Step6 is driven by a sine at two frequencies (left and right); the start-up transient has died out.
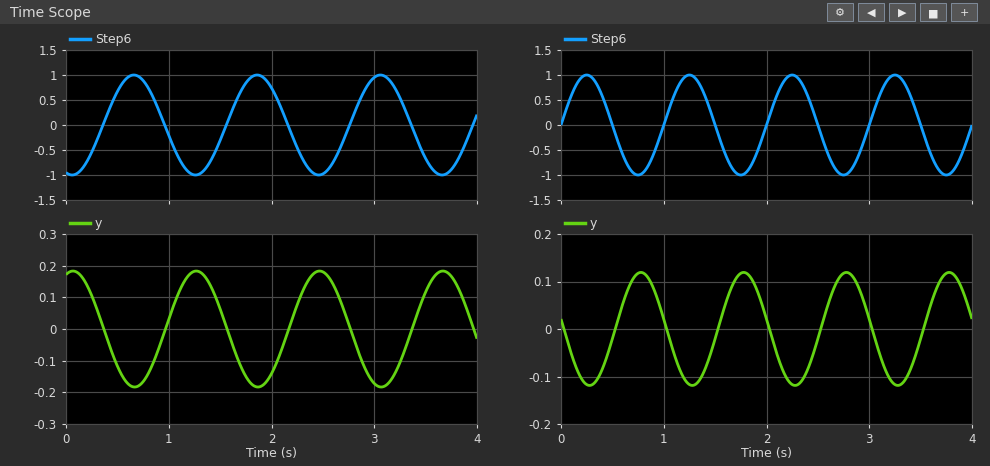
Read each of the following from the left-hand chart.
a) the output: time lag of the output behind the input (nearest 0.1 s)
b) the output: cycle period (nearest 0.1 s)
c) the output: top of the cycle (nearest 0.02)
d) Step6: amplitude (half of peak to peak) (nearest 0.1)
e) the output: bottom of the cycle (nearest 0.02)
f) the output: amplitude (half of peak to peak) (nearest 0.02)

0.6 s
1.2 s
0.18
1.0
-0.18
0.18
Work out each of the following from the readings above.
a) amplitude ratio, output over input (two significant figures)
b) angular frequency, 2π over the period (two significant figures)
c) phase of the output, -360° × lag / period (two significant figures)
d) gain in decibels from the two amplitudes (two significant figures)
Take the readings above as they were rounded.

0.18
5.2 rad/s
-180°
-15 dB
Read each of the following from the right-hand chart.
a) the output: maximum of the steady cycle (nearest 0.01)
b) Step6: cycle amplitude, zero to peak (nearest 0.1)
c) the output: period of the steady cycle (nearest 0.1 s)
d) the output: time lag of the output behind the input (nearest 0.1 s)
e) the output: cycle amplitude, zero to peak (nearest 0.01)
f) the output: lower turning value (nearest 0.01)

0.12
1.0
1.0 s
0.5 s
0.12
-0.12
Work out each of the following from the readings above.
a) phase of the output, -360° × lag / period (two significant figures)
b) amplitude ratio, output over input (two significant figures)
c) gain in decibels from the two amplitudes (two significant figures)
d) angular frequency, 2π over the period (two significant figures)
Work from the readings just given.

-180°
0.12
-18 dB
6.3 rad/s
